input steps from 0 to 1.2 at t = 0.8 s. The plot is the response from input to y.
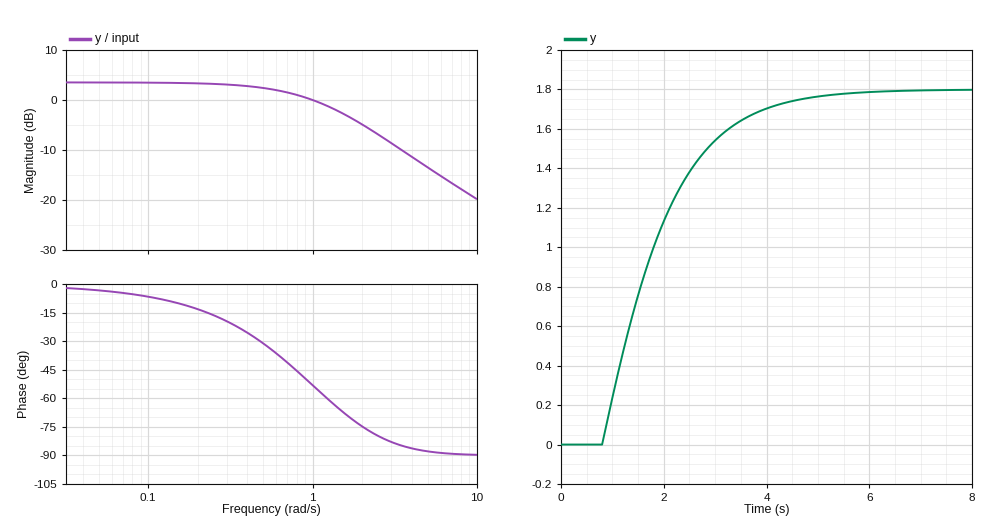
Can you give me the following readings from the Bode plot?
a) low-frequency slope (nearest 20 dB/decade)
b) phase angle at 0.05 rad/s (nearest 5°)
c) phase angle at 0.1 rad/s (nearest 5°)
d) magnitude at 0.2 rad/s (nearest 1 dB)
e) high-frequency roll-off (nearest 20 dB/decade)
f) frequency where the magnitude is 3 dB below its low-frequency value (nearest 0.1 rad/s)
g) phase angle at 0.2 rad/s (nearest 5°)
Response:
0 dB/decade
-5°
-5°
3 dB
-20 dB/decade
0.9 rad/s
-15°
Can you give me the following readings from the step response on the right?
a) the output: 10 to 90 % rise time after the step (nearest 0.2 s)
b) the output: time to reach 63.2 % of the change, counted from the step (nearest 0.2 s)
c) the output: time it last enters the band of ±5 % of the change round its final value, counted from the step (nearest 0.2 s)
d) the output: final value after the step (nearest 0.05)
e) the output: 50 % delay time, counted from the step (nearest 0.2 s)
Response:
2.4 s
1.2 s
3.2 s
1.80
0.8 s
